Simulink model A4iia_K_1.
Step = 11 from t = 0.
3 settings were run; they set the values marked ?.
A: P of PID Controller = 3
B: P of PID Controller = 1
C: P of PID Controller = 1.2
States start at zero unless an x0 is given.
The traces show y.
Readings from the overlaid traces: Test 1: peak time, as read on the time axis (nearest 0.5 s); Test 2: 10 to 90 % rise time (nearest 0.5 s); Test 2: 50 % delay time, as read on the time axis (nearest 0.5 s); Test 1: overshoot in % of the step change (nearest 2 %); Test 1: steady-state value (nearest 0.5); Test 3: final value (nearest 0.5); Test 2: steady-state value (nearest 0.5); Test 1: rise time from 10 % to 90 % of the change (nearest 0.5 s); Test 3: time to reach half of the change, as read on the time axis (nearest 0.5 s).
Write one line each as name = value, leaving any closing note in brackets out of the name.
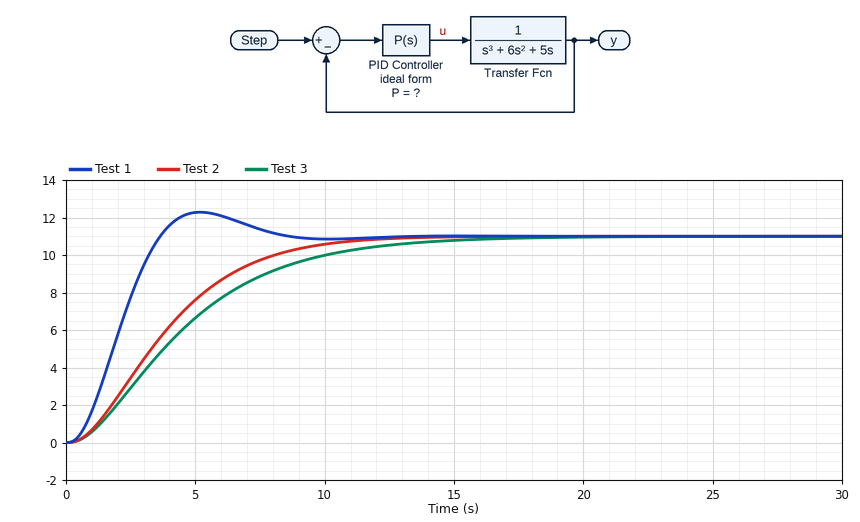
Test 1: peak time, as read on the time axis = 5.0 s
Test 2: 10 to 90 % rise time = 6.5 s
Test 2: 50 % delay time, as read on the time axis = 3.5 s
Test 1: overshoot in % of the step change = 12 %
Test 1: steady-state value = 11.0
Test 3: final value = 11.0
Test 2: steady-state value = 11.0
Test 1: rise time from 10 % to 90 % of the change = 2.5 s
Test 3: time to reach half of the change, as read on the time axis = 4.0 s
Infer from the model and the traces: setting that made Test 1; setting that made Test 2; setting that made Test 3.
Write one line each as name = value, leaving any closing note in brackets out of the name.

setting that made Test 1 = A
setting that made Test 2 = C
setting that made Test 3 = B
